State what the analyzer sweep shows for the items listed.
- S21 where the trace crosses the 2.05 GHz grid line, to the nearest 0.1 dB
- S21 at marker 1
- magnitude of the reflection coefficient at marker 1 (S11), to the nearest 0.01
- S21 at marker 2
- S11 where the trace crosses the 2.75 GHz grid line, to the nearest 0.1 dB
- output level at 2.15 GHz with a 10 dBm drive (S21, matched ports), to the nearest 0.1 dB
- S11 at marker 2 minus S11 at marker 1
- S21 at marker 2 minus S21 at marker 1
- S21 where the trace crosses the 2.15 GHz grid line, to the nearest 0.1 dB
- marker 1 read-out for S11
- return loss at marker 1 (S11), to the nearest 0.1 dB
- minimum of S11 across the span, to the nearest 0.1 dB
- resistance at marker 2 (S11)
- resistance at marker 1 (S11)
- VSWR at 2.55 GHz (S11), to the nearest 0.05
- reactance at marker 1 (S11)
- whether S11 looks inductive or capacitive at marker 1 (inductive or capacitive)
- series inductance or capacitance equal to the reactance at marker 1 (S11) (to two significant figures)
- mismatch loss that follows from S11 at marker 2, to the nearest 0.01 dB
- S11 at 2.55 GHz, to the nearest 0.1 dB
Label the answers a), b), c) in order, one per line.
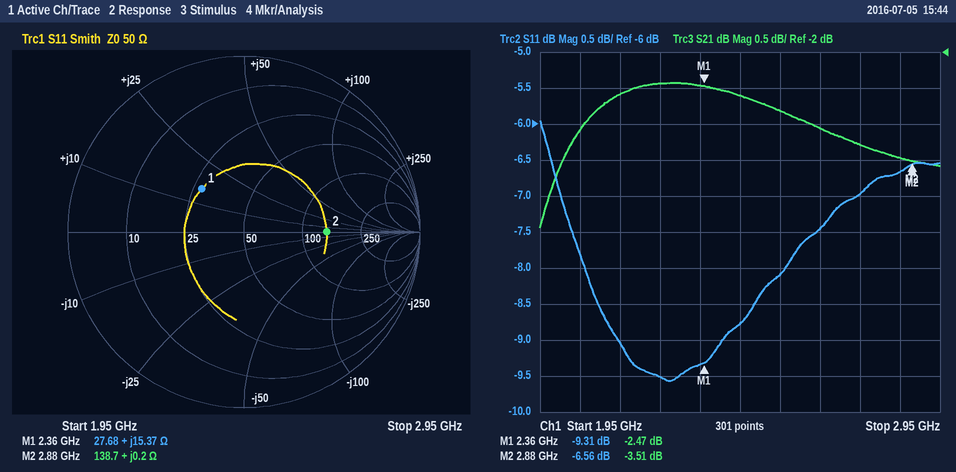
a) -3.1 dB
b) -2.47 dB
c) 0.34
d) -3.51 dB
e) -7.0 dB
f) 7.4 dBm
g) 2.75 dB
h) -1.04 dB
i) -2.6 dB
j) -9.31 dB
k) 9.3 dB
l) -9.6 dB
m) 138.7 Ω
n) 27.68 Ω
o) 2.30
p) +15.37 Ω
q) inductive
r) 1.0 nH
s) 1.08 dB
t) -8.1 dB
